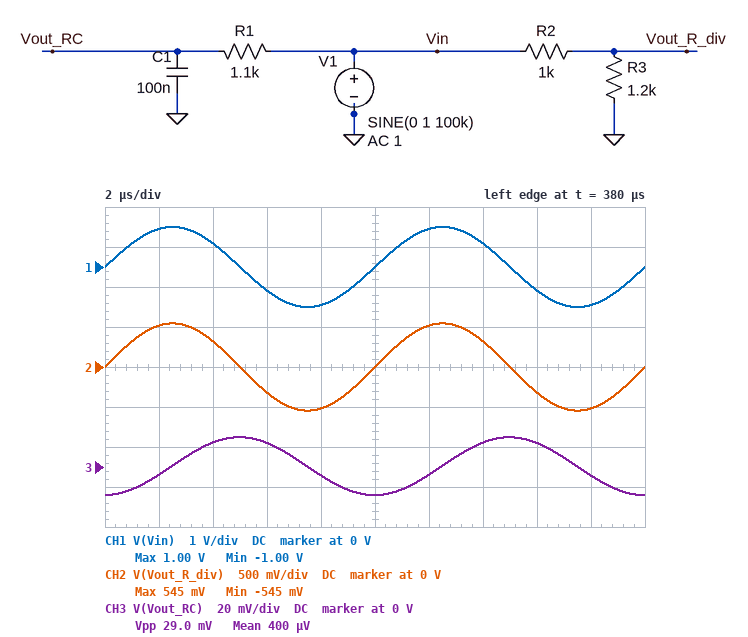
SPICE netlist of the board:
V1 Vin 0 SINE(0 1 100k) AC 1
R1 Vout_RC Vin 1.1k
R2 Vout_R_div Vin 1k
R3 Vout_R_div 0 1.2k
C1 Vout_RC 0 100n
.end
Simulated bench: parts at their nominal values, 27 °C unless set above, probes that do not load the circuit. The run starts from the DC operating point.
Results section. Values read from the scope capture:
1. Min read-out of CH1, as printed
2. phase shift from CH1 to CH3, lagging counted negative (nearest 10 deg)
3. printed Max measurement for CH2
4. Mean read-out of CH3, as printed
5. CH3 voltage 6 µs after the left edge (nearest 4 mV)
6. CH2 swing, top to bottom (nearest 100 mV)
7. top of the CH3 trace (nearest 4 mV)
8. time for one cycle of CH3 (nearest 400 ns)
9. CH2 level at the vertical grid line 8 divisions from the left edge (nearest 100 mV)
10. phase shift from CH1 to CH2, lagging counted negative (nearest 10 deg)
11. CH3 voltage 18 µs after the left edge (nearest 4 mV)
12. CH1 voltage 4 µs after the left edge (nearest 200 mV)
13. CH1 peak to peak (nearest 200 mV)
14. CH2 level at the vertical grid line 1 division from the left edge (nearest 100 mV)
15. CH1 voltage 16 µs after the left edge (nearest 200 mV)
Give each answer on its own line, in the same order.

-1.00 V
-90 deg
545 mV
400 µV
12 mV
1.1 V
16 mV
10.0 µs
-300 mV
0 deg
-4 mV
600 mV
2.0 V
500 mV
-600 mV
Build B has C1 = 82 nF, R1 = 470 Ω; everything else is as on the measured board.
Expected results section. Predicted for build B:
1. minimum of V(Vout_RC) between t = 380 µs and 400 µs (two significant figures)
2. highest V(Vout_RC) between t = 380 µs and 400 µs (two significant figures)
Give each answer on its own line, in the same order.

-41 mV
41 mV
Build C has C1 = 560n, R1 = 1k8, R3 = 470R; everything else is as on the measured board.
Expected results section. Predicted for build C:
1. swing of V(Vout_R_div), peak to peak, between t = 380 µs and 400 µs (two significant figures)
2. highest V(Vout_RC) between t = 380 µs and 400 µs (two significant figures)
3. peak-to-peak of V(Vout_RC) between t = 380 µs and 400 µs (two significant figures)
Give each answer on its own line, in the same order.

640 mV
2.7 mV
3.2 mV
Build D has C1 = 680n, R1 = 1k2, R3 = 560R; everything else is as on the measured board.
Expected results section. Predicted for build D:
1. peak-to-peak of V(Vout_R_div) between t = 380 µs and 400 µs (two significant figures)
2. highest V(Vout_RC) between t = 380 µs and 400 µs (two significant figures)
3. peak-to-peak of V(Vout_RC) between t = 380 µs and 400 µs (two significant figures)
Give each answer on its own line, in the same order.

720 mV
3.2 mV
3.9 mV
